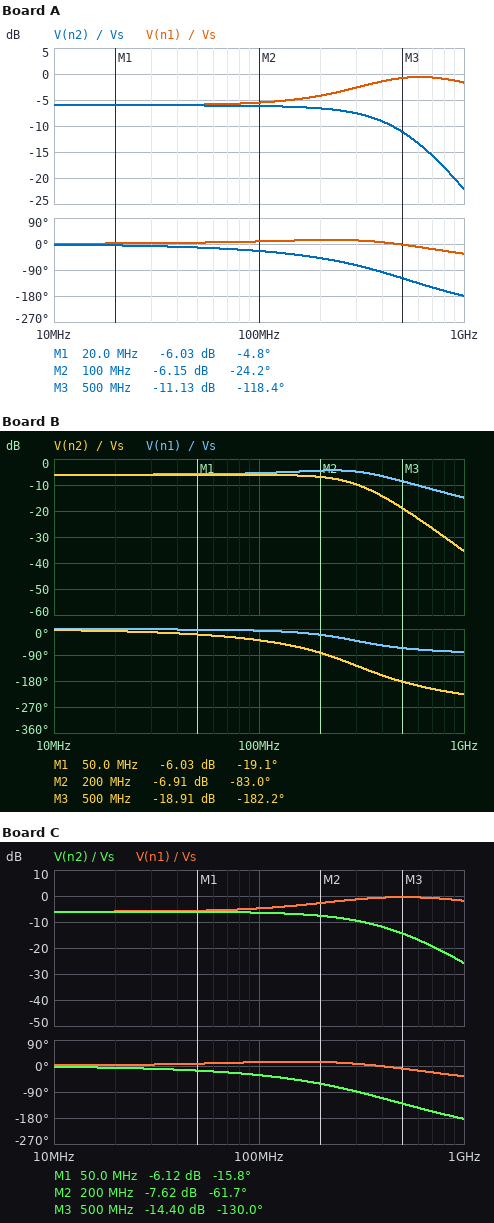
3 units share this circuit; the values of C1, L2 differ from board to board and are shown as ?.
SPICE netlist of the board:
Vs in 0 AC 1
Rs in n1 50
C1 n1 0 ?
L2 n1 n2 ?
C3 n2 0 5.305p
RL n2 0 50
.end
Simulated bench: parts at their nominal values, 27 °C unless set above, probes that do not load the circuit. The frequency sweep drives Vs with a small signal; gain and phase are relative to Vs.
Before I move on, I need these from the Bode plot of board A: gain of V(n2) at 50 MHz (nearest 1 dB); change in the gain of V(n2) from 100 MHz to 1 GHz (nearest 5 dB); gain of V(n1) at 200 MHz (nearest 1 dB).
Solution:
-6 dB
-15 dB
-4 dB
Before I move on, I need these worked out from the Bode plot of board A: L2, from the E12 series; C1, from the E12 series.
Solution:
47 nH
2.7 pF
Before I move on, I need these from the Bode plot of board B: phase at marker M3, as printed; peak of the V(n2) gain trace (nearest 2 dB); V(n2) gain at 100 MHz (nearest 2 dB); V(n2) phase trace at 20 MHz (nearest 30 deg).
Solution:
-182.2 deg
-6 dB
-6 dB
0 deg
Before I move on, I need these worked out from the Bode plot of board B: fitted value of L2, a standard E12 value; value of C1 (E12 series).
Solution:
47 nH
18 pF
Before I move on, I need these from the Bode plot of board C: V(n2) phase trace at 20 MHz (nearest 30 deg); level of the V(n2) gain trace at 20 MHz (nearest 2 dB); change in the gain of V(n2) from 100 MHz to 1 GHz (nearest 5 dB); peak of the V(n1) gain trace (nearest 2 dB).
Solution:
0 deg
-6 dB
-20 dB
0 dB
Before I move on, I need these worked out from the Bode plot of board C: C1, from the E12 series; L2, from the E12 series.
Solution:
2.7 pF
68 nH
